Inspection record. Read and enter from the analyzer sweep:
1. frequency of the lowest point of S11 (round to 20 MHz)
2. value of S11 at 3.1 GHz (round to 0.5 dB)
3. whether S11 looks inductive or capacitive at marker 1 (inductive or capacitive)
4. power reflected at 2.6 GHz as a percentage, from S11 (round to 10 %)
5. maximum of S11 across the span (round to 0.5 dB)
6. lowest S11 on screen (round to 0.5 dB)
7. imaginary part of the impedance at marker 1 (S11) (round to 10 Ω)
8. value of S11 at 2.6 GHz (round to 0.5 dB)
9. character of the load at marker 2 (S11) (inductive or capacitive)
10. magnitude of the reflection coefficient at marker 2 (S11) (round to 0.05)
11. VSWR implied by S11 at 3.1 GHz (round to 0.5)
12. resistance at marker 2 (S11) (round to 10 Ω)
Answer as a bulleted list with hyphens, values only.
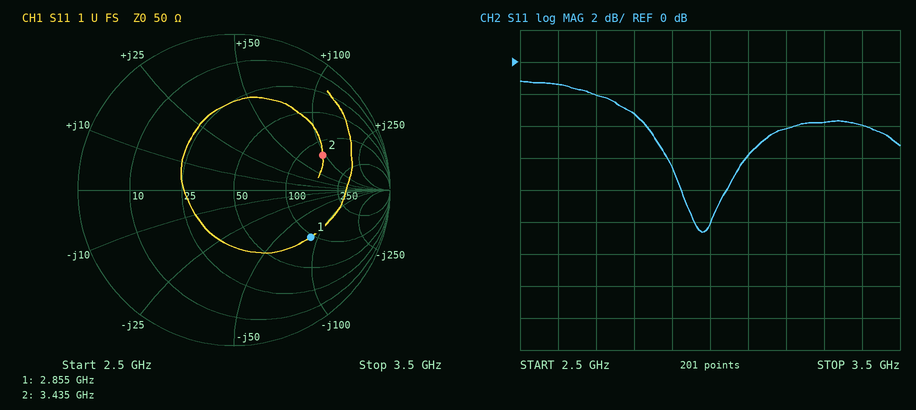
- 2.98 GHz
- -6.0 dB
- capacitive
- 70 %
- -1.0 dB
- -10.5 dB
- -90 Ω
- -1.5 dB
- inductive
- 0.60
- 3.0
- 130 Ω
